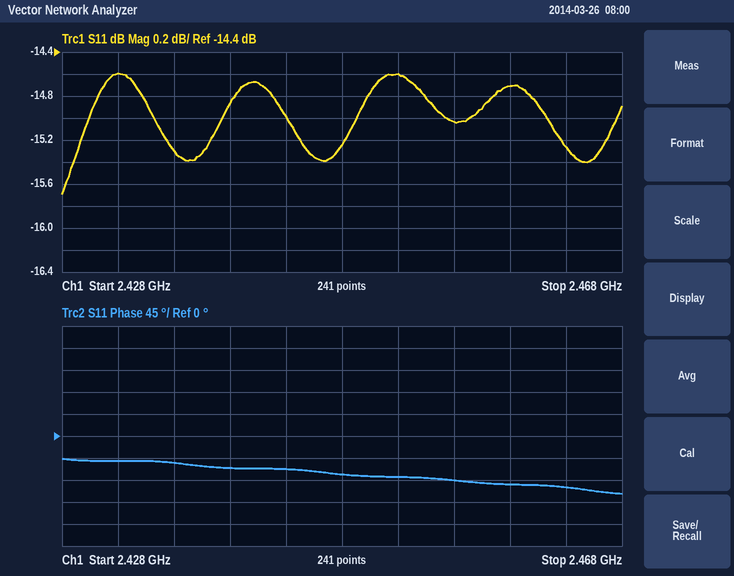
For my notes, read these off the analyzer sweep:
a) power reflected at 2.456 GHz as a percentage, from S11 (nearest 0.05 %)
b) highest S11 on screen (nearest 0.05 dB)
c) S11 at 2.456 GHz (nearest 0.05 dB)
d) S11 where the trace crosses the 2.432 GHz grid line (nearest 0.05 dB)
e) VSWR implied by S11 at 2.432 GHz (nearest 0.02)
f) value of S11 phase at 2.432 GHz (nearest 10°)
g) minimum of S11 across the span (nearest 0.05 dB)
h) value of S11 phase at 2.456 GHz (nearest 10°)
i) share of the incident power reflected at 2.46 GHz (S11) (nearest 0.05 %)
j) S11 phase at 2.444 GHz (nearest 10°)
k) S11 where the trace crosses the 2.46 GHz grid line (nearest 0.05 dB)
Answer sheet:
3.15 %
-14.60 dB
-15.05 dB
-14.60 dB
1.46
-50°
-15.70 dB
-90°
3.40 %
-70°
-14.70 dB
